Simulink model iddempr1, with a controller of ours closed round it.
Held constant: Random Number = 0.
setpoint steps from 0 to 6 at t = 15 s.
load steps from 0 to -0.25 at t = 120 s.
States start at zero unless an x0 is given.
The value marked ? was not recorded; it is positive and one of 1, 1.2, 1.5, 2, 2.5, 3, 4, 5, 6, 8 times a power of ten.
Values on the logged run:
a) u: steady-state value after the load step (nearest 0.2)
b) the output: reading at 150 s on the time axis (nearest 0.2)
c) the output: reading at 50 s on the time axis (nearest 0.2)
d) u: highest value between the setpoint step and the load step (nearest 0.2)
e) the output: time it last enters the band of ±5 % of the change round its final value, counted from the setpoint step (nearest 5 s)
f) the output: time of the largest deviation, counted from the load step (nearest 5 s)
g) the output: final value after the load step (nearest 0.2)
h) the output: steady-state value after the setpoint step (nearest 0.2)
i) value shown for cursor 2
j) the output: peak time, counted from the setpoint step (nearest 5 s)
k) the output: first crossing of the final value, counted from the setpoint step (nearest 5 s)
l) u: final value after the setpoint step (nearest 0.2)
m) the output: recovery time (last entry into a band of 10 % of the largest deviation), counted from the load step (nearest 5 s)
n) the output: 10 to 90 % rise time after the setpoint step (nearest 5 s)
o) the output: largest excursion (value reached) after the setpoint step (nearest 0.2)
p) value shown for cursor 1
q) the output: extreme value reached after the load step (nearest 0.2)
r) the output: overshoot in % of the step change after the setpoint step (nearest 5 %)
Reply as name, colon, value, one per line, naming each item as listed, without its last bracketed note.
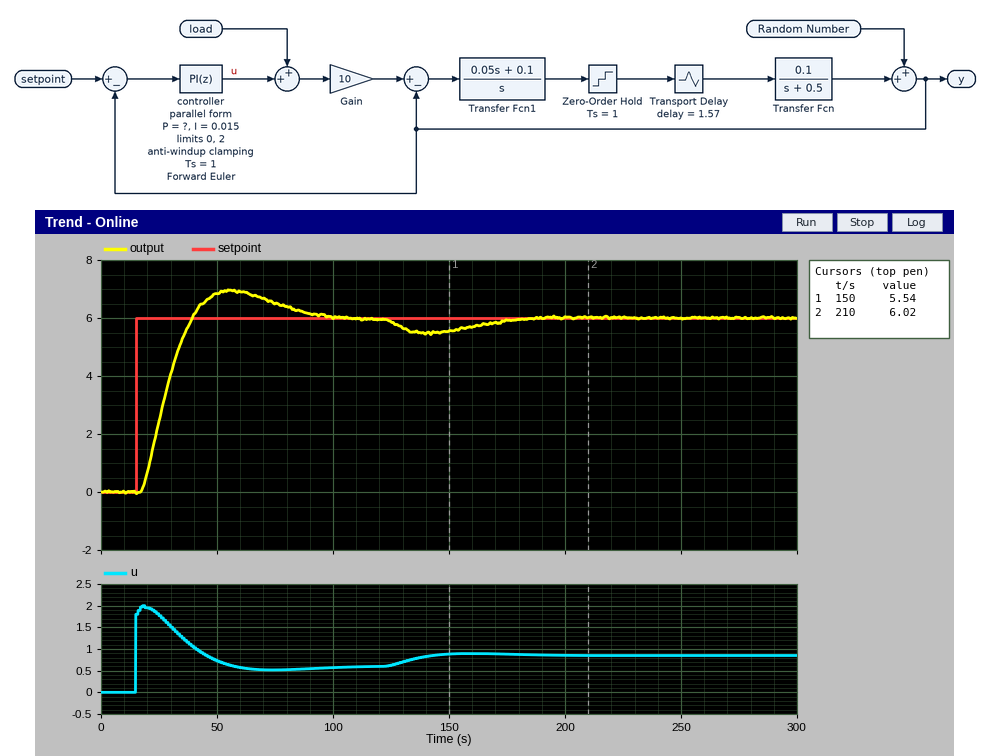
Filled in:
u: steady-state value after the load step: 0.8
the output: reading at 150 s on the time axis: 5.6
the output: reading at 50 s on the time axis: 6.8
u: highest value between the setpoint step and the load step: 2.0
the output: time it last enters the band of ±5 % of the change round its final value, counted from the setpoint step: 70 s
the output: time of the largest deviation, counted from the load step: 20 s
the output: final value after the load step: 6.0
the output: steady-state value after the setpoint step: 6.0
value shown for cursor 2: 6.02
the output: peak time, counted from the setpoint step: 40 s
the output: first crossing of the final value, counted from the setpoint step: 25 s
u: final value after the setpoint step: 0.6
the output: recovery time (last entry into a band of 10 % of the largest deviation), counted from the load step: 60 s
the output: 10 to 90 % rise time after the setpoint step: 15 s
the output: largest excursion (value reached) after the setpoint step: 7.0
value shown for cursor 1: 5.54
the output: extreme value reached after the load step: 5.4
the output: overshoot in % of the step change after the setpoint step: 15 %
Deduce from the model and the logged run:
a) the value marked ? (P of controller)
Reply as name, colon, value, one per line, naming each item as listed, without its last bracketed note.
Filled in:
the value marked ?: 0.3
